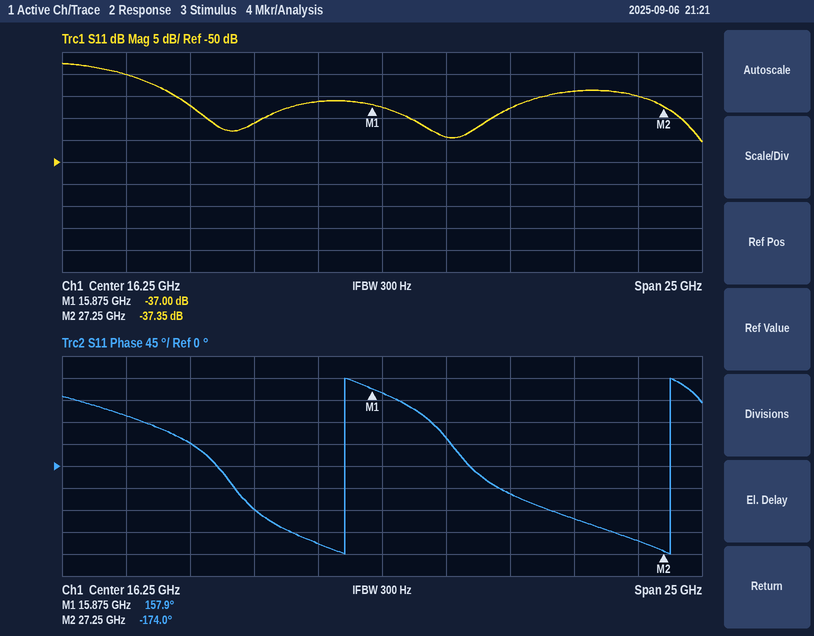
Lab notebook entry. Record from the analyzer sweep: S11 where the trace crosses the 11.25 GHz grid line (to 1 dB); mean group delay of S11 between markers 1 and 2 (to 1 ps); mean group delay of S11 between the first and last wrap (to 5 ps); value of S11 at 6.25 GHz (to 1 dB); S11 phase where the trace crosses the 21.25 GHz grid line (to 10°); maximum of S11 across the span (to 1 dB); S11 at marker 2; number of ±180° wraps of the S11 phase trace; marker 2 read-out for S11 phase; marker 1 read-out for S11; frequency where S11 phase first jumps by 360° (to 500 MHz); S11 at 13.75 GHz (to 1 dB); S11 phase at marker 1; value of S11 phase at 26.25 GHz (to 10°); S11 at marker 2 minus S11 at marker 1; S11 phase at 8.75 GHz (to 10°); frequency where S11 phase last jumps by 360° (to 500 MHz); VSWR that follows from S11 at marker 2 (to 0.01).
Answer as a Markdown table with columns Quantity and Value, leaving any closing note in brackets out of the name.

| Quantity | Value |
|---|---|
| S11 where the trace crosses the 11.25 GHz grid line | -41 dB |
| mean group delay of S11 between markers 1 and 2 | 81 ps |
| mean group delay of S11 between the first and last wrap | 80 ps |
| value of S11 at 6.25 GHz | -30 dB |
| S11 phase where the trace crosses the 21.25 GHz grid line | -60° |
| maximum of S11 across the span | -28 dB |
| S11 at marker 2 | -37.35 dB |
| number of ±180° wraps of the S11 phase trace | 2 |
| marker 2 read-out for S11 phase | -174.0° |
| marker 1 read-out for S11 | -37.00 dB |
| frequency where S11 phase first jumps by 360° | 15.0 GHz |
| S11 at 13.75 GHz | -36 dB |
| S11 phase at marker 1 | 157.9° |
| value of S11 phase at 26.25 GHz | -150° |
| S11 at marker 2 minus S11 at marker 1 | -0.35 dB |
| S11 phase at 8.75 GHz | 50° |
| frequency where S11 phase last jumps by 360° | 27.5 GHz |
| VSWR that follows from S11 at marker 2 | 1.03 |
